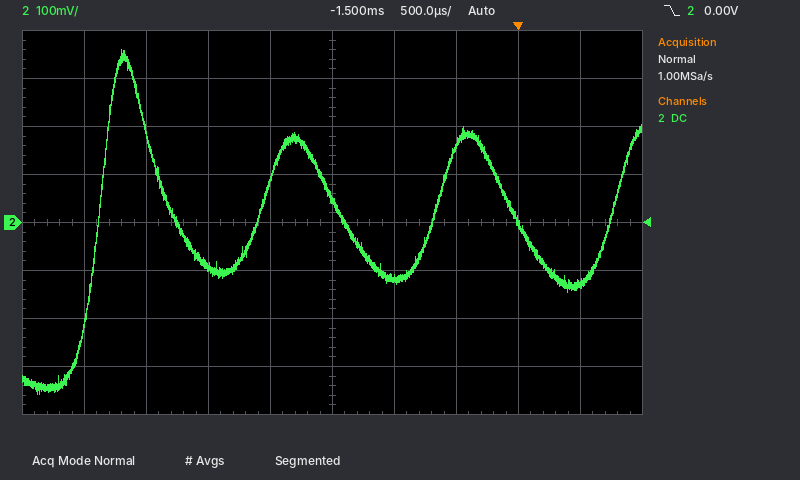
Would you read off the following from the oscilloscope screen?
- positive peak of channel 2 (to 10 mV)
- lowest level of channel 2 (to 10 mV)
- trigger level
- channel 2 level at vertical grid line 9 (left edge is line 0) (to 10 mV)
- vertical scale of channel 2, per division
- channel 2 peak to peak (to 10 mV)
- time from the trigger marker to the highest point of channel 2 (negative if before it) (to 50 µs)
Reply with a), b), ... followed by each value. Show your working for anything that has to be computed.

a) 360 mV
b) -360 mV
c) 0.00 V
d) -130 mV
e) 100 mV
f) 360 mV − (-360 mV) = 720 mV
g) -3.20 ms
